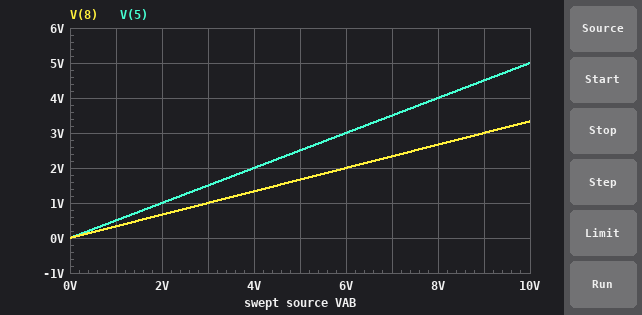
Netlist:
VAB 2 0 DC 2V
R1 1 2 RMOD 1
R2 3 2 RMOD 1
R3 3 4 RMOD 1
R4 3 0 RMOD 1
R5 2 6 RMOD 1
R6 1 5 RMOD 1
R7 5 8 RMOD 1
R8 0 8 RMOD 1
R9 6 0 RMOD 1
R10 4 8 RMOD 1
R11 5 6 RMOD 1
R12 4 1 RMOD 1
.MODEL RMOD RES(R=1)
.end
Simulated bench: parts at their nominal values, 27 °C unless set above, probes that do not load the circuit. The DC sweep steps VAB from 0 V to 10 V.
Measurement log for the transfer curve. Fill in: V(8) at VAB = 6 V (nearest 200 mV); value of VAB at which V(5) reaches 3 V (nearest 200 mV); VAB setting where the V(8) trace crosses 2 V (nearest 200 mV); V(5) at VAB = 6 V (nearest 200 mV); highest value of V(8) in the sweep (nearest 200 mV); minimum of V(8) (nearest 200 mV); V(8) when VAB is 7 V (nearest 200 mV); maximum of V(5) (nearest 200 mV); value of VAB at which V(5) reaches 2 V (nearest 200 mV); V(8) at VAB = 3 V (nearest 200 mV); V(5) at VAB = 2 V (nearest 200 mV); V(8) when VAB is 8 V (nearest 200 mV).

2.0 V
6.0 V
6.0 V
3.0 V
3.4 V
0 V
2.4 V
5.0 V
4.0 V
1.0 V
1.0 V
2.6 V
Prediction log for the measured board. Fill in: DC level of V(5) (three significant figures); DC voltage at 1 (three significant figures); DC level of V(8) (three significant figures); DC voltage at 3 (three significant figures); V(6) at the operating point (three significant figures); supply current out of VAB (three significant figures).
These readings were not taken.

1.00 V
1.33 V
667 mV
1.00 V
1.00 V
2.67 A
